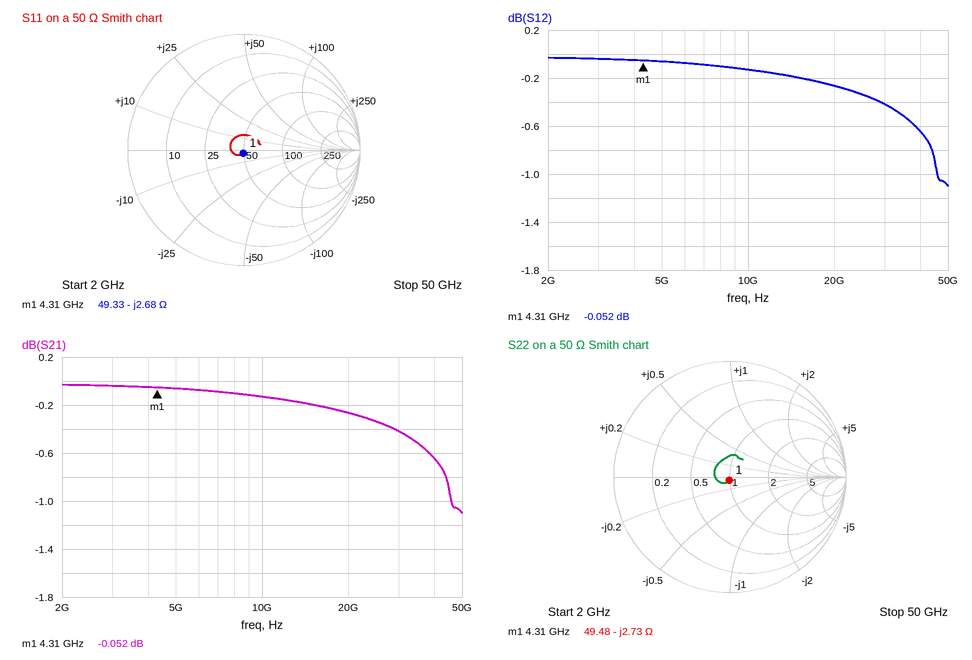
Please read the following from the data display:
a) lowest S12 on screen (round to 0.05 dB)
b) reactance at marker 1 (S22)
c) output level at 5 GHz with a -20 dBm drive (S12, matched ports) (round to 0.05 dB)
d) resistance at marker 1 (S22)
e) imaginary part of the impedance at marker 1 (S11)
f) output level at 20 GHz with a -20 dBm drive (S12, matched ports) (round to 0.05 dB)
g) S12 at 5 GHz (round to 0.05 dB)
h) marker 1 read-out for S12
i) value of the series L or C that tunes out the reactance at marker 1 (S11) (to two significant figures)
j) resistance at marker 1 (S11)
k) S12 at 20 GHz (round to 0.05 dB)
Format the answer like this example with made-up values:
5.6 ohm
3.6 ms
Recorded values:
-1.10 dB
-2.73 Ω
-20.05 dBm
49.48 Ω
-2.68 Ω
-20.25 dBm
-0.05 dB
-0.052 dB
99 pH
49.33 Ω
-0.25 dB
